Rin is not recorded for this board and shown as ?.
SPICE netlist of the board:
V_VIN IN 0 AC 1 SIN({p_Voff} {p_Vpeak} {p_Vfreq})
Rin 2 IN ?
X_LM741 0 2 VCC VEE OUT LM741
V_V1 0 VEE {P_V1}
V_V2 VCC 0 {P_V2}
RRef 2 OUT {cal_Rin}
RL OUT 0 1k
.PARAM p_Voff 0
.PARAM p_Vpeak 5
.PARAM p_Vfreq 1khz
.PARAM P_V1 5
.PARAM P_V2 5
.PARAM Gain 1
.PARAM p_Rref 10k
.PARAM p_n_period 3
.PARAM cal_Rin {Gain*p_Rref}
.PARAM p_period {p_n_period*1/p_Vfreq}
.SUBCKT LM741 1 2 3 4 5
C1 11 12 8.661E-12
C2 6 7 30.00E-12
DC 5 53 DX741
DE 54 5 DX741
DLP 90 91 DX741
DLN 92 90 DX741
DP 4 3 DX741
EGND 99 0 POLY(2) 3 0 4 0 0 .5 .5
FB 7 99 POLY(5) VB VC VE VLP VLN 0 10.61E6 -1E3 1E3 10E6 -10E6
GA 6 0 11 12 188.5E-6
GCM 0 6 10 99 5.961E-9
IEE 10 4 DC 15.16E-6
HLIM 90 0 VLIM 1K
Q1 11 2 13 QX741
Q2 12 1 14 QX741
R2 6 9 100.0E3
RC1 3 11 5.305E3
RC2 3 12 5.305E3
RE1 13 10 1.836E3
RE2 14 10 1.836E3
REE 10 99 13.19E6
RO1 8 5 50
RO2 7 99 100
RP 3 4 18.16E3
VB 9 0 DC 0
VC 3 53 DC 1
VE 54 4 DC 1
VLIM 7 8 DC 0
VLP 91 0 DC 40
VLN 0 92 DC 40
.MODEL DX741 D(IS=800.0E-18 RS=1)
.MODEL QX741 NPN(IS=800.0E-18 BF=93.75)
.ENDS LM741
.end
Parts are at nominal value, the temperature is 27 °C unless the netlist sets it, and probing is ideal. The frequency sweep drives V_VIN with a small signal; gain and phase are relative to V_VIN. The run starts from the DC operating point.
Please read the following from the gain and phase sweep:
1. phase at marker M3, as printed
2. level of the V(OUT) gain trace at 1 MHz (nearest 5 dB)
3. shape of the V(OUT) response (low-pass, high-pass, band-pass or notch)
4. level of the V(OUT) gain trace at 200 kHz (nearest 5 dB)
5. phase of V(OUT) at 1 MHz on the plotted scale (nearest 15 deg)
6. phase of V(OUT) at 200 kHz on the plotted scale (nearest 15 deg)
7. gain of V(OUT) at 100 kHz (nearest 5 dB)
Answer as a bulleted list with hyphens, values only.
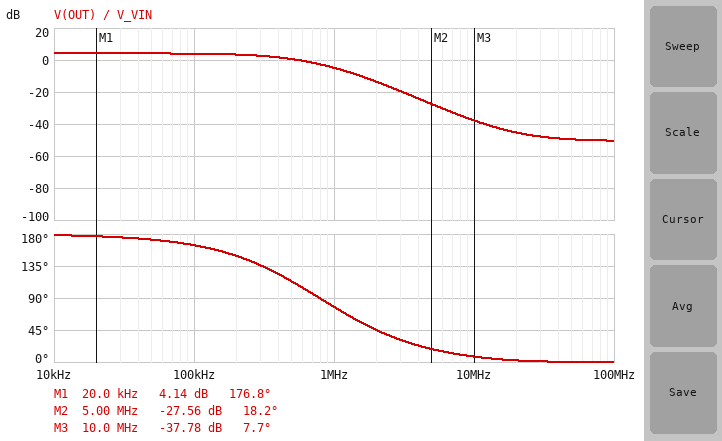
- 7.7 deg
- -5 dB
- low-pass
- 5 dB
- 75 deg
- 150 deg
- 5 dB
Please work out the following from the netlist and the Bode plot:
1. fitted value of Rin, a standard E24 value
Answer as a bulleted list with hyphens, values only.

- 6.2 kΩ
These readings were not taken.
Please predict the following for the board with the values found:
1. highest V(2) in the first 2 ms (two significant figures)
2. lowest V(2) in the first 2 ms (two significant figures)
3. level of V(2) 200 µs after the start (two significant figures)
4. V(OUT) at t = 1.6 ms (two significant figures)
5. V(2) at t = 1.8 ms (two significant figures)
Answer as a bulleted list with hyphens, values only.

- 1.2 V
- -1.2 V
- 1.1 V
- 4.7 V
- -1.1 V
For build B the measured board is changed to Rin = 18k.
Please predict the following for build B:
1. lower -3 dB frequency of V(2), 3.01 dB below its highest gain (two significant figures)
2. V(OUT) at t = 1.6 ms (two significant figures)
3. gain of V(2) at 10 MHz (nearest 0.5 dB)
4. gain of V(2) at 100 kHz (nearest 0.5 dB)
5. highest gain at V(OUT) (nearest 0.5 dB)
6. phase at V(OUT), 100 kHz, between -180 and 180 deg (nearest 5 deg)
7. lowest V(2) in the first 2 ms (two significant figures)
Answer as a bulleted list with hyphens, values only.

- 570 kHz
- 1.6 V
- -9.0 dB
- -24.5 dB
- -5.0 dB
- 170 deg
- -2.9 mV
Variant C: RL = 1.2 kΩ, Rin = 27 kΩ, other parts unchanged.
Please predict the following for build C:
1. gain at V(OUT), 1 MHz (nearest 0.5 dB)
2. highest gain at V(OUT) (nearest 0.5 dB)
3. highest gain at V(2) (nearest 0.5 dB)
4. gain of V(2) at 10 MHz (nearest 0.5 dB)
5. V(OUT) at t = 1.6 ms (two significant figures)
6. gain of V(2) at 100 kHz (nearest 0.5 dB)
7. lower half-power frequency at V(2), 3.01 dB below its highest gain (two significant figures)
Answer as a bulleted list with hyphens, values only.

- -12.0 dB
- -8.5 dB
- -9.5 dB
- -11.5 dB
- 1.1 V
- -28.0 dB
- 640 kHz
